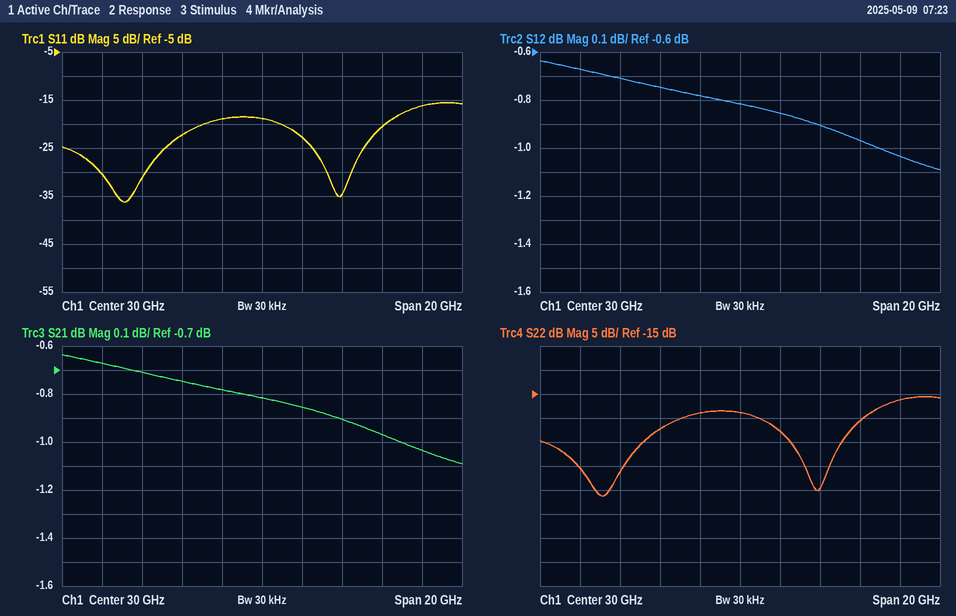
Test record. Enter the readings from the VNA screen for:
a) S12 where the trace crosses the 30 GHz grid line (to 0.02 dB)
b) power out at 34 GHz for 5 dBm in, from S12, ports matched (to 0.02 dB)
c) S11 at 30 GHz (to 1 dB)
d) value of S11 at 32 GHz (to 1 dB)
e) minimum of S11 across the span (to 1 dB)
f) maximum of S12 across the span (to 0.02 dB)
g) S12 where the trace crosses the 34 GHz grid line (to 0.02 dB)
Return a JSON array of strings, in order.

["-0.82 dB", "4.10 dBm", "-19 dB", "-23 dB", "-36 dB", "-0.64 dB", "-0.90 dB"]
